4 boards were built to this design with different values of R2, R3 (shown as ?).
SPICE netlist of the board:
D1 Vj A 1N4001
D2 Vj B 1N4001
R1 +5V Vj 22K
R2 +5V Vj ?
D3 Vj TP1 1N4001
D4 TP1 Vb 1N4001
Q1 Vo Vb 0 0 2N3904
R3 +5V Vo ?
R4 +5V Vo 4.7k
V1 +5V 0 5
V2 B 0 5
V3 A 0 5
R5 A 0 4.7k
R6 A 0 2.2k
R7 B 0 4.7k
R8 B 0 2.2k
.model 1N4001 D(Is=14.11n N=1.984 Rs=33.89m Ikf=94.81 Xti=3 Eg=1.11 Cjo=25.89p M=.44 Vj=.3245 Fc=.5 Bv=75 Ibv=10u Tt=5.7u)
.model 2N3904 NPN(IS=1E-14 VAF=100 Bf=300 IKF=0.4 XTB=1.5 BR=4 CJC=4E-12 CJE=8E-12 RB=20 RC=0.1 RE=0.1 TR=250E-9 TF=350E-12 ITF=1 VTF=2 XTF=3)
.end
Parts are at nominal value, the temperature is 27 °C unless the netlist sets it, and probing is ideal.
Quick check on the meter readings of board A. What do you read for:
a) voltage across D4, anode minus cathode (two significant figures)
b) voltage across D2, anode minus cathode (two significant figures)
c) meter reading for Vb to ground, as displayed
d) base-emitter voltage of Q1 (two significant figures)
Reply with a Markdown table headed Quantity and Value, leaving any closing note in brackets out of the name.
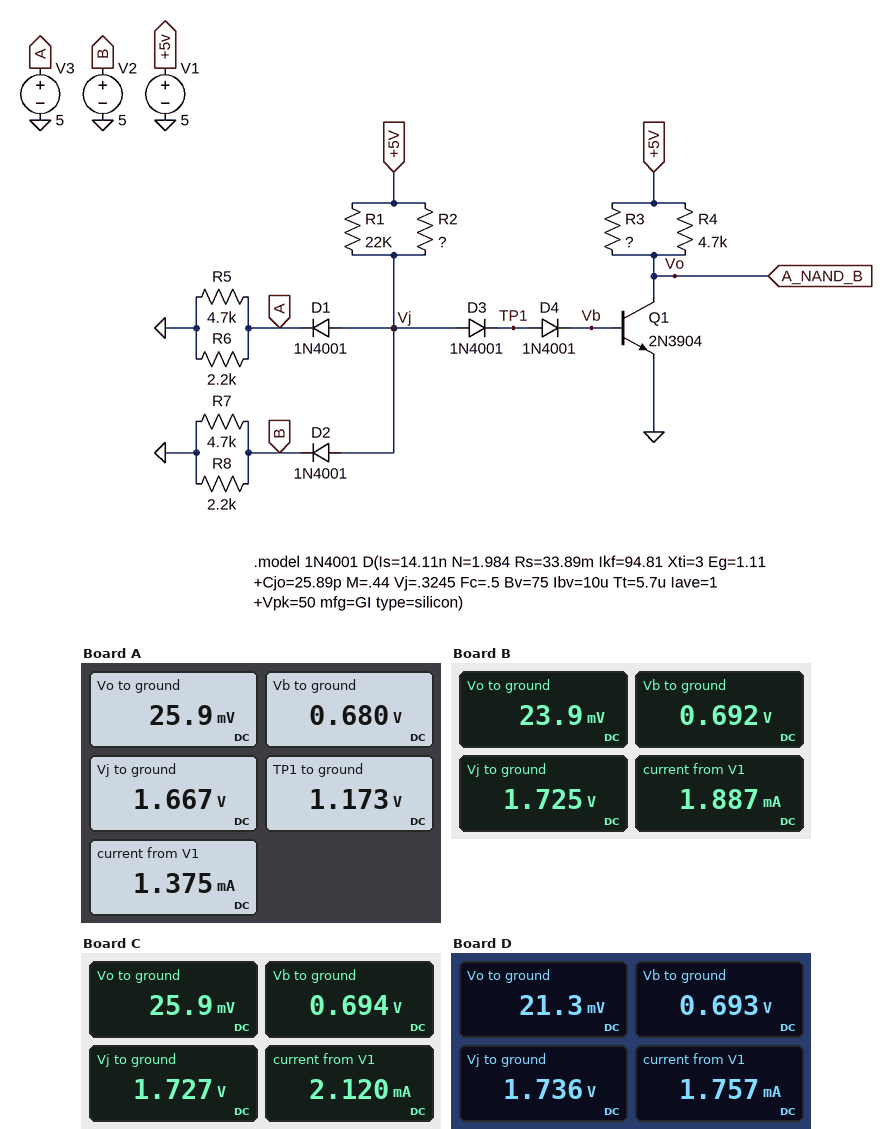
| Quantity | Value |
|---|---|
| voltage across D4, anode minus cathode | 490 mV |
| voltage across D2, anode minus cathode | -3.3 V |
| meter reading for Vb to ground, as displayed | 0.680 V |
| base-emitter voltage of Q1 | 680 mV |
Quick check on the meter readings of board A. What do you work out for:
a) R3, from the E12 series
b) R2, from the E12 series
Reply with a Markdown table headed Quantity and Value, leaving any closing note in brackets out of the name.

| Quantity | Value |
|---|---|
| R3, from the E12 series | 47 kΩ |
| R2, from the E12 series | 56 kΩ |
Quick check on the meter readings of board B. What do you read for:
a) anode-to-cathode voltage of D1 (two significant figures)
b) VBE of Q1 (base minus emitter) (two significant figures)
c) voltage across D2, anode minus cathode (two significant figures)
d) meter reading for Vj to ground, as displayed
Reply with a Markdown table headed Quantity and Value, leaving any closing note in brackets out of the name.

| Quantity | Value |
|---|---|
| anode-to-cathode voltage of D1 | -3.3 V |
| VBE of Q1 (base minus emitter) | 690 mV |
| voltage across D2, anode minus cathode | -3.3 V |
| meter reading for Vj to ground, as displayed | 1.725 V |
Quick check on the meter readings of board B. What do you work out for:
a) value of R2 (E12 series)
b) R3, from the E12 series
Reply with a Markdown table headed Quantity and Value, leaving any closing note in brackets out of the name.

| Quantity | Value |
|---|---|
| value of R2 | 18 kΩ |
| R3, from the E12 series | 10 kΩ |
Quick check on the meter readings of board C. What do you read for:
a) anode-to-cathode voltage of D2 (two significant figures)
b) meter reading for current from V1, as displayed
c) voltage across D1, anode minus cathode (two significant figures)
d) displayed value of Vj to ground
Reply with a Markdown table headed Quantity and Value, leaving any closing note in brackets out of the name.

| Quantity | Value |
|---|---|
| anode-to-cathode voltage of D2 | -3.3 V |
| meter reading for current from V1, as displayed | 2.120 mA |
| voltage across D1, anode minus cathode | -3.3 V |
| displayed value of Vj to ground | 1.727 V |
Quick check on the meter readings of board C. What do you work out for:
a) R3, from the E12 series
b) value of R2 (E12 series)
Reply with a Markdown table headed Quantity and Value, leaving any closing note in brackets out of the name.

| Quantity | Value |
|---|---|
| R3, from the E12 series | 6.8 kΩ |
| value of R2 | 18 kΩ |
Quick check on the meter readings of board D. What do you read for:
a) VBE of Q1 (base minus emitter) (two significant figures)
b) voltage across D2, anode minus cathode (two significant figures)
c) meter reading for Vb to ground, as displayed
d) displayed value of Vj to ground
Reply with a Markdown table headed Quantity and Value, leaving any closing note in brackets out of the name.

| Quantity | Value |
|---|---|
| VBE of Q1 (base minus emitter) | 690 mV |
| voltage across D2, anode minus cathode | -3.3 V |
| meter reading for Vb to ground, as displayed | 0.693 V |
| displayed value of Vj to ground | 1.736 V |
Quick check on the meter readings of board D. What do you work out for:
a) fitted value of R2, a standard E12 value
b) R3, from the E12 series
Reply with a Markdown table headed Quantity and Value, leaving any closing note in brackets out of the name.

| Quantity | Value |
|---|---|
| fitted value of R2, a standard E12 value | 15 kΩ |
| R3, from the E12 series | 15 kΩ |
